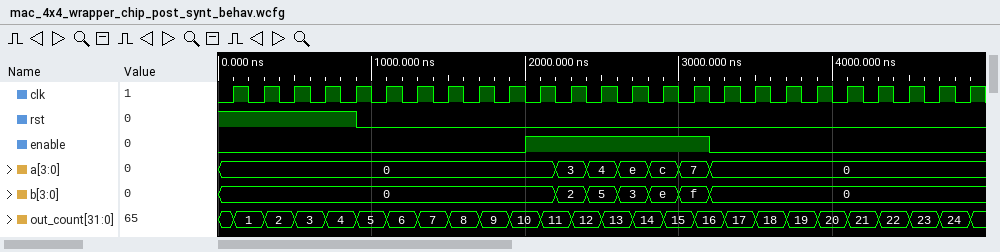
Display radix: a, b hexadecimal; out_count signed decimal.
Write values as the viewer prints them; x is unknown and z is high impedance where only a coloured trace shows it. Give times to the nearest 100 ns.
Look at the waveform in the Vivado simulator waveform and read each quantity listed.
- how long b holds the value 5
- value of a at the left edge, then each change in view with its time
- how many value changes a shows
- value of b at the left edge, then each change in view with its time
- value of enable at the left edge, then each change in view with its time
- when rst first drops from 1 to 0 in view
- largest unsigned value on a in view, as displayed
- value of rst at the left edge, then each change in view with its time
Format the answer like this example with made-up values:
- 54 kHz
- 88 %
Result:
- 200 ns
- 0, 3 at 2200 ns, 4 at 2400 ns, e at 2600 ns, c at 2800 ns, 7 at 3000 ns, 0 at 3200 ns
- 6
- 0, 2 at 2200 ns, 5 at 2400 ns, 3 at 2600 ns, e at 2800 ns, f at 3000 ns, 0 at 3200 ns
- 0, 1 at 2000 ns, 0 at 3200 ns
- 900 ns
- e
- 1, 0 at 900 ns
